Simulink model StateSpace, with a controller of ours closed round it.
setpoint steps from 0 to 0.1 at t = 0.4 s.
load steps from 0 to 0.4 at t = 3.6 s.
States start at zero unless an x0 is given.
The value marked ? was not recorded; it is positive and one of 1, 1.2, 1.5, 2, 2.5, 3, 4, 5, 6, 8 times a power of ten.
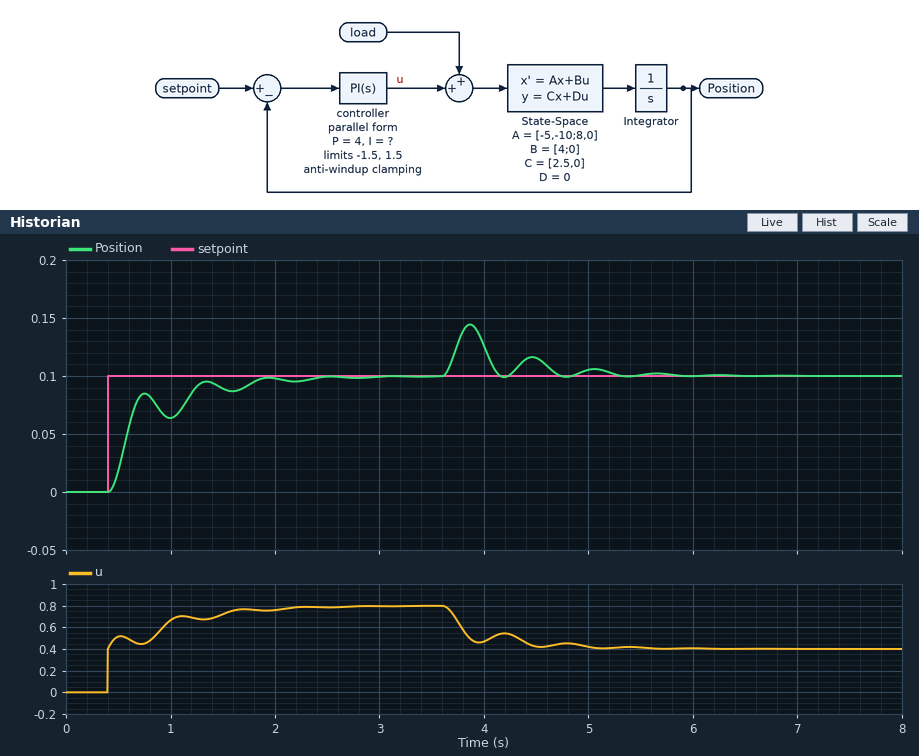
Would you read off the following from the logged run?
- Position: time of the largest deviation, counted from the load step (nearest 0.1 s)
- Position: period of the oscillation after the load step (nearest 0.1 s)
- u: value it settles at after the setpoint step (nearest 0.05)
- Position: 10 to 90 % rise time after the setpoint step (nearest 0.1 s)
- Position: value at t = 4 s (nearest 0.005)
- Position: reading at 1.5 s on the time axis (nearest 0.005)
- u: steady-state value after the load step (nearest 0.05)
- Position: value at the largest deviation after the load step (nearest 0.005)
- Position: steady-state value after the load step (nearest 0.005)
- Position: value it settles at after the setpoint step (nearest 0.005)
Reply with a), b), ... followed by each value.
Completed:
a) 0.3 s
b) 0.6 s
c) 0.80
d) 0.8 s
e) 0.125
f) 0.090
g) 0.40
h) 0.145
i) 0.100
j) 0.100
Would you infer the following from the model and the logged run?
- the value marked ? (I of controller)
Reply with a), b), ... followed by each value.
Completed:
a) 20
